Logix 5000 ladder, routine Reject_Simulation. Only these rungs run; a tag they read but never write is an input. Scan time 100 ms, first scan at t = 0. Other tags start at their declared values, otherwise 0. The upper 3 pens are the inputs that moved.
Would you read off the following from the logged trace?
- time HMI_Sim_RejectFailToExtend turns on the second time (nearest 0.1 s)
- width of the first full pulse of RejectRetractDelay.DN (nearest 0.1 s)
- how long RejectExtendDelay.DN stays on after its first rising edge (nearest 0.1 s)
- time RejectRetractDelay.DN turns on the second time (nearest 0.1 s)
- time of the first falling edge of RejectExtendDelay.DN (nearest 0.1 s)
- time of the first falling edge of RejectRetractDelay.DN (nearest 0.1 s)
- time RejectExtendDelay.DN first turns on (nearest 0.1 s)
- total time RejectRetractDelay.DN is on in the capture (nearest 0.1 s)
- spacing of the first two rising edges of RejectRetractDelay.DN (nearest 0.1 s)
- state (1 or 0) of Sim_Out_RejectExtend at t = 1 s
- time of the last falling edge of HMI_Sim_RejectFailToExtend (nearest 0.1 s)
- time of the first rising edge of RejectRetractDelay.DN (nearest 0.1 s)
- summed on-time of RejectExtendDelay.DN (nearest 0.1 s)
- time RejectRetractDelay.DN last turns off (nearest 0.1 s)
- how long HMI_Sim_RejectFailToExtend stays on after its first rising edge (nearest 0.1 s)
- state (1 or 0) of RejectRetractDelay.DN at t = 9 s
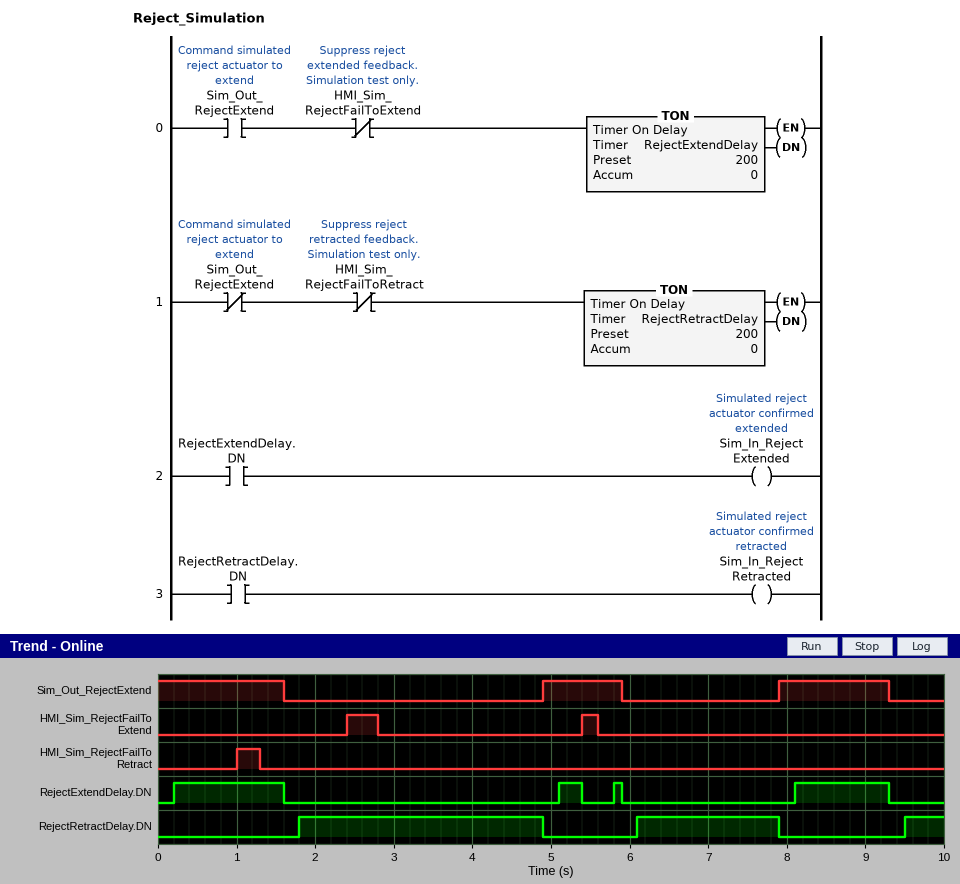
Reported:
5.4 s
3.1 s
1.4 s
6.1 s
1.6 s
4.9 s
0.2 s
5.4 s
4.3 s
1
5.6 s
1.8 s
3.0 s
7.9 s
0.4 s
0
